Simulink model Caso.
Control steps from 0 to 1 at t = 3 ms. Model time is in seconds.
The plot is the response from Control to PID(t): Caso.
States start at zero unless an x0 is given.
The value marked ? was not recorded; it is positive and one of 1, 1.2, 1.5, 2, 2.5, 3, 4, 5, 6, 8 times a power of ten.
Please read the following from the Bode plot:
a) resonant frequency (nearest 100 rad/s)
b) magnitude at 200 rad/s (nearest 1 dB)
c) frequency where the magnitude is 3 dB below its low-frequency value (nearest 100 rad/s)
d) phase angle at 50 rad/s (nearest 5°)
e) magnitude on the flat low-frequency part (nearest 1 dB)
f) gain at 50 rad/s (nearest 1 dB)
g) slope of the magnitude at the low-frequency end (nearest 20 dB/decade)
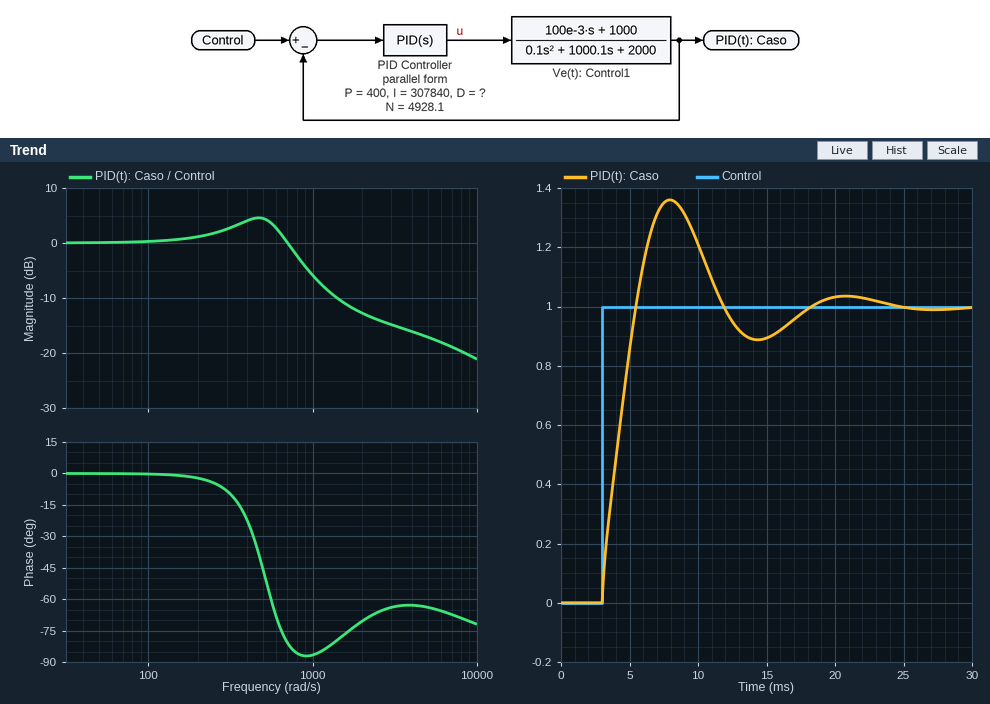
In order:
500 rad/s
1 dB
800 rad/s
0°
0 dB
0 dB
0 dB/decade
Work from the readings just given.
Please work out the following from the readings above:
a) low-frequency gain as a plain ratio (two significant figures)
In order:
1.0
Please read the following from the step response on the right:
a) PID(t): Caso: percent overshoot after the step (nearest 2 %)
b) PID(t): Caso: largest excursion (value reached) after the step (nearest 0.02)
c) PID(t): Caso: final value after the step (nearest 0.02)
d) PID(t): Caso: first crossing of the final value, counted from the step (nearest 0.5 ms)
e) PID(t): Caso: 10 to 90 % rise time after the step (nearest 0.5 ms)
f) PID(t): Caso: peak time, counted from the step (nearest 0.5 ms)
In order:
36 %
1.36
1.00
2.5 ms
2.0 ms
5.0 ms
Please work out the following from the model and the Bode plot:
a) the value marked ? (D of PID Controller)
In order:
0.12
